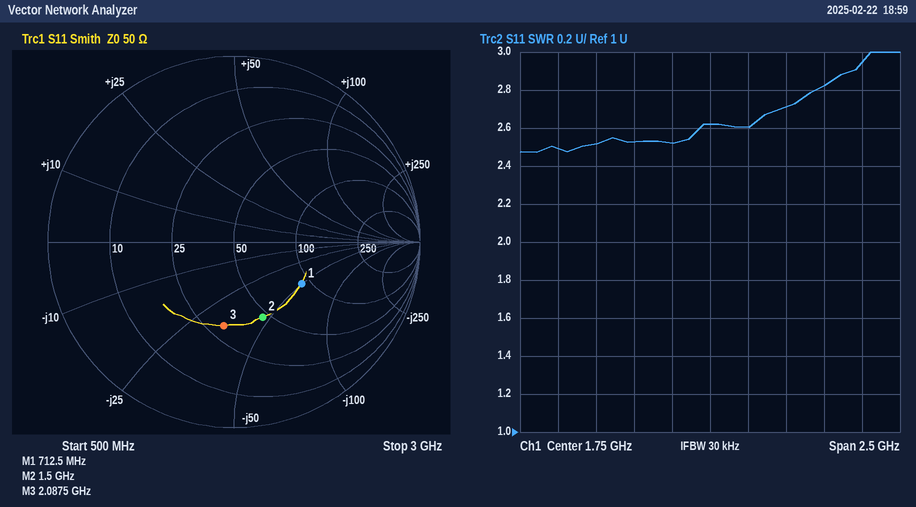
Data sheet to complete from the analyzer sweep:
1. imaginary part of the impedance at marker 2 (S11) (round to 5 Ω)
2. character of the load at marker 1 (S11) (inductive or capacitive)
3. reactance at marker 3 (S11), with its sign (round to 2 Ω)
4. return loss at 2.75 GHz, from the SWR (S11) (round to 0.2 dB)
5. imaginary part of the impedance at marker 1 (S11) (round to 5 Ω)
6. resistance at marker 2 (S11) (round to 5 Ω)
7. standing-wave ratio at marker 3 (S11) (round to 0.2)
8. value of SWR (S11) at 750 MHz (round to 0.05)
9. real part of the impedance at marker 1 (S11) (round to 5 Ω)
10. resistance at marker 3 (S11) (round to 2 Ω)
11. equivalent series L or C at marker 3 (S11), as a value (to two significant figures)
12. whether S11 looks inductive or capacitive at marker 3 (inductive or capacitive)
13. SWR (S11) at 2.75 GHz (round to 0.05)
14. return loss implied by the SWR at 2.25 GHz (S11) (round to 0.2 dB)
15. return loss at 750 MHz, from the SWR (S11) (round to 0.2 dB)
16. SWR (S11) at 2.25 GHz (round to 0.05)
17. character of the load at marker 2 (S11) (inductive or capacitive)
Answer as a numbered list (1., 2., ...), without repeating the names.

1. -45 Ω
2. capacitive
3. -34 Ω
4. 6.2 dB
5. -50 Ω
6. 45 Ω
7. 2.6
8. 2.50
9. 90 Ω
10. 30 Ω
11. 2.2 pF
12. capacitive
13. 2.95
14. 6.8 dB
15. 7.4 dB
16. 2.70
17. capacitive
